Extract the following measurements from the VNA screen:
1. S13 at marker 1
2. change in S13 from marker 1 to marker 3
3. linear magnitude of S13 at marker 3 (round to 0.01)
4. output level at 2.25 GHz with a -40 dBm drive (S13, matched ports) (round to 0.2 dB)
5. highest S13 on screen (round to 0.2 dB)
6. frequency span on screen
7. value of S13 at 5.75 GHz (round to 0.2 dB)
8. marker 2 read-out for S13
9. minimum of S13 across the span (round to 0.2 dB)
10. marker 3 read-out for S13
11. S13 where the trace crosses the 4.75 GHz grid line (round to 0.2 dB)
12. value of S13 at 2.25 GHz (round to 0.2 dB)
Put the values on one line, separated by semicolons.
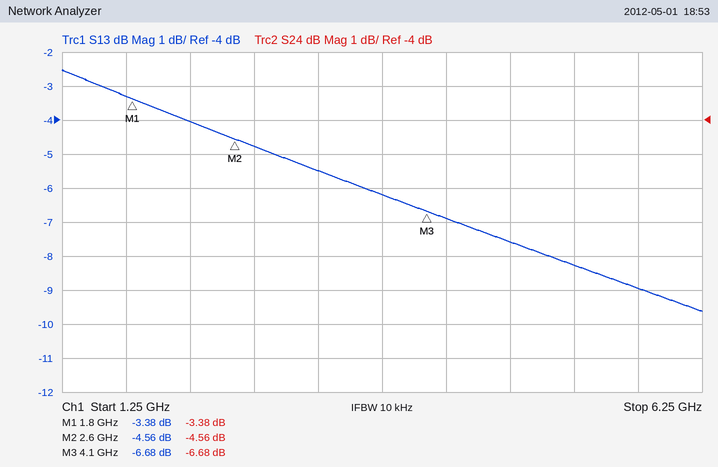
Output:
-3.38 dB; -3.30 dB; 0.46; -44.0 dBm; -2.6 dB; 5 GHz; -9.0 dB; -4.56 dB; -9.6 dB; -6.68 dB; -7.6 dB; -4.0 dB
